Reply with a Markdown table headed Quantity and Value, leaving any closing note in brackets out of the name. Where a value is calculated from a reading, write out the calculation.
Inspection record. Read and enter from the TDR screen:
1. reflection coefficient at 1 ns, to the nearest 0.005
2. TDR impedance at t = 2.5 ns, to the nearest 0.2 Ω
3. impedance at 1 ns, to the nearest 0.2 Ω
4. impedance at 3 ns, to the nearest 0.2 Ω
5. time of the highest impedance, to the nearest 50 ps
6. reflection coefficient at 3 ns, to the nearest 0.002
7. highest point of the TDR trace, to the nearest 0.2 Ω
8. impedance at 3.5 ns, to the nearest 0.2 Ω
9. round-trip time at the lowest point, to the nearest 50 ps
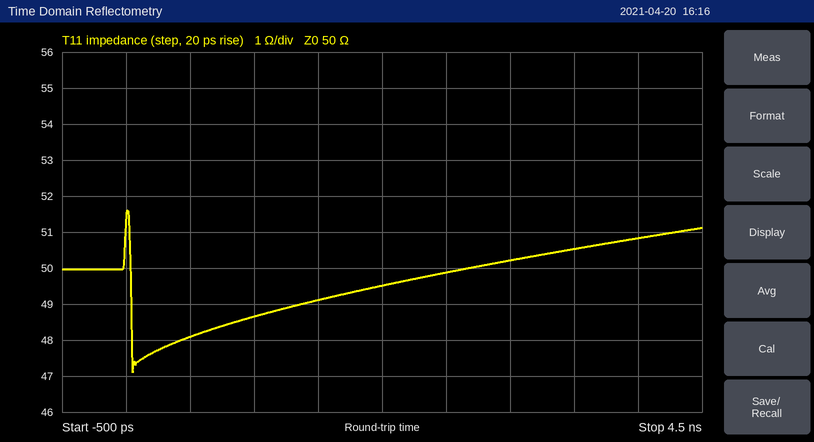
| Quantity | Value |
|---|---|
| reflection coefficient at 1 ns, to the nearest 0.005 | (48.6 − 50)/(48.6 + 50) ≈ -0.0142, so -0.015 to the nearest 0.005 |
| TDR impedance at t = 2.5 ns, to the nearest 0.2 Ω | 49.8 Ω |
| impedance at 1 ns, to the nearest 0.2 Ω | 48.6 Ω |
| impedance at 3 ns, to the nearest 0.2 Ω | 50.2 Ω |
| time of the highest impedance, to the nearest 50 ps | 0 ps |
| reflection coefficient at 3 ns, to the nearest 0.002 | (50.2 − 50)/(50.2 + 50) ≈ +0.002 |
| highest point of the TDR trace, to the nearest 0.2 Ω | 51.6 Ω |
| impedance at 3.5 ns, to the nearest 0.2 Ω | 50.6 Ω |
| round-trip time at the lowest point, to the nearest 50 ps | 50 ps |
